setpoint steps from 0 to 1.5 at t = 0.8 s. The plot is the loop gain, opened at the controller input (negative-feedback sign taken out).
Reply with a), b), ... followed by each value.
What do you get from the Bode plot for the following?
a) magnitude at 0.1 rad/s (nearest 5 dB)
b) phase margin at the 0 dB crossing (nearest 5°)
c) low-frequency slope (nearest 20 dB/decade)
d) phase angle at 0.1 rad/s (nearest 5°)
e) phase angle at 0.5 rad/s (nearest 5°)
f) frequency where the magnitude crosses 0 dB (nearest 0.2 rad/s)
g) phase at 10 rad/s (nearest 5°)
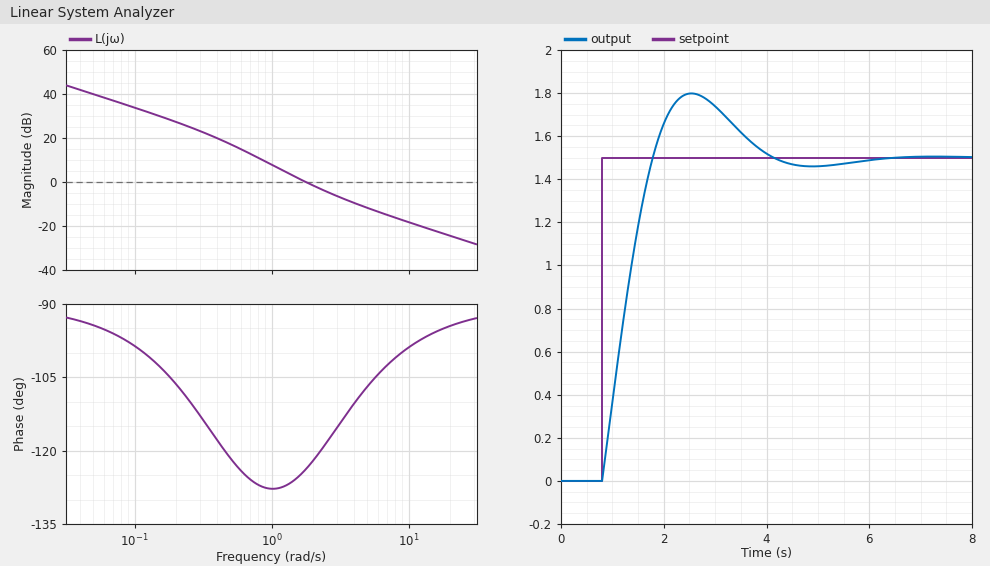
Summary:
a) 35 dB
b) 55°
c) -20 dB/decade
d) -100°
e) -120°
f) 1.8 rad/s
g) -100°
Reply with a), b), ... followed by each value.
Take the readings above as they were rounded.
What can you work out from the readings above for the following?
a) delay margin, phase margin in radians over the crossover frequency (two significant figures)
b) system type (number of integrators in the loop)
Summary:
a) 0.53 s
b) 1
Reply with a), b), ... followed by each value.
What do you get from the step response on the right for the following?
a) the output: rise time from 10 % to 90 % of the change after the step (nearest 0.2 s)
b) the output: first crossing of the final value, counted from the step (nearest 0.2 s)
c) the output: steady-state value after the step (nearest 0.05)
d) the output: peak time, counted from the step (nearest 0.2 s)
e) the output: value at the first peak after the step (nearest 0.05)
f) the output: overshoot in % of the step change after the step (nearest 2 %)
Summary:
a) 0.8 s
b) 1.0 s
c) 1.50
d) 1.8 s
e) 1.80
f) 20 %
